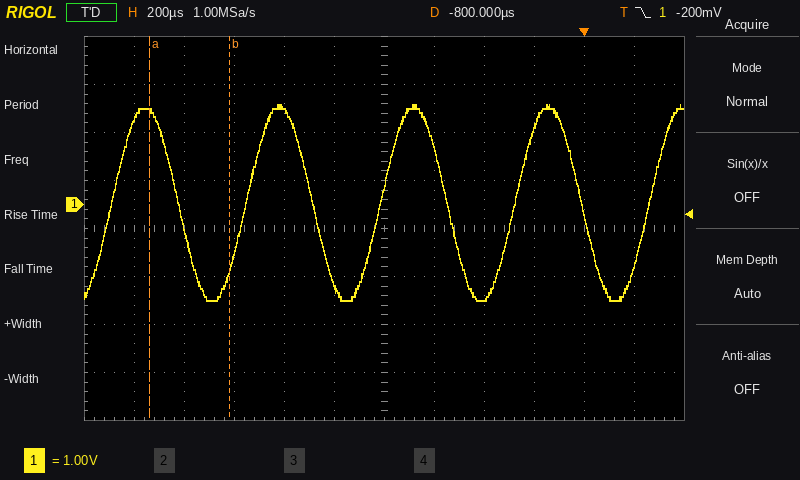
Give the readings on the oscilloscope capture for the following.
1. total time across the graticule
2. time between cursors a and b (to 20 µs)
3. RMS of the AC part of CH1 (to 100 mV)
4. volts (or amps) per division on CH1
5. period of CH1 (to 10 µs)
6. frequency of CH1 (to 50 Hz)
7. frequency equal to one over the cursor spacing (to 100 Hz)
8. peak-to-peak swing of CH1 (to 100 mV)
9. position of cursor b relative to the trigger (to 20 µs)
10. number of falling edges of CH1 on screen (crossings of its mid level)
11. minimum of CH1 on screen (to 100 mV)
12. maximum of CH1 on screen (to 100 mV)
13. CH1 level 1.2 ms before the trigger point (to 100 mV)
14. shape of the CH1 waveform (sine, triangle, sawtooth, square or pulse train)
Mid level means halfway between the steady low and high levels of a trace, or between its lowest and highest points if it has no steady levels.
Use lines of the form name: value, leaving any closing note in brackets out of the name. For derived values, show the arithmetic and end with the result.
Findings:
total time across the graticule: 2.4 ms
time between cursors a and b: 320 µs
RMS of the AC part of CH1: 4.1 V / (2√2) ≈ 1.4 V
volts (or amps) per division on CH1: 1 V
period of CH1: 540 µs
frequency of CH1: 1 / 540 µs ≈ 1.85 kHz
frequency equal to one over the cursor spacing: 1 / 320 µs ≈ 3.1 kHz
peak-to-peak swing of CH1: 2.1 V − (-2.0 V) = 4.1 V
position of cursor b relative to the trigger: -1.42 ms
number of falling edges of CH1 on screen: 4
minimum of CH1 on screen: -2.0 V
maximum of CH1 on screen: 2.1 V
CH1 level 1.2 ms before the trigger point: 2.0 V
shape of the CH1 waveform: sine
